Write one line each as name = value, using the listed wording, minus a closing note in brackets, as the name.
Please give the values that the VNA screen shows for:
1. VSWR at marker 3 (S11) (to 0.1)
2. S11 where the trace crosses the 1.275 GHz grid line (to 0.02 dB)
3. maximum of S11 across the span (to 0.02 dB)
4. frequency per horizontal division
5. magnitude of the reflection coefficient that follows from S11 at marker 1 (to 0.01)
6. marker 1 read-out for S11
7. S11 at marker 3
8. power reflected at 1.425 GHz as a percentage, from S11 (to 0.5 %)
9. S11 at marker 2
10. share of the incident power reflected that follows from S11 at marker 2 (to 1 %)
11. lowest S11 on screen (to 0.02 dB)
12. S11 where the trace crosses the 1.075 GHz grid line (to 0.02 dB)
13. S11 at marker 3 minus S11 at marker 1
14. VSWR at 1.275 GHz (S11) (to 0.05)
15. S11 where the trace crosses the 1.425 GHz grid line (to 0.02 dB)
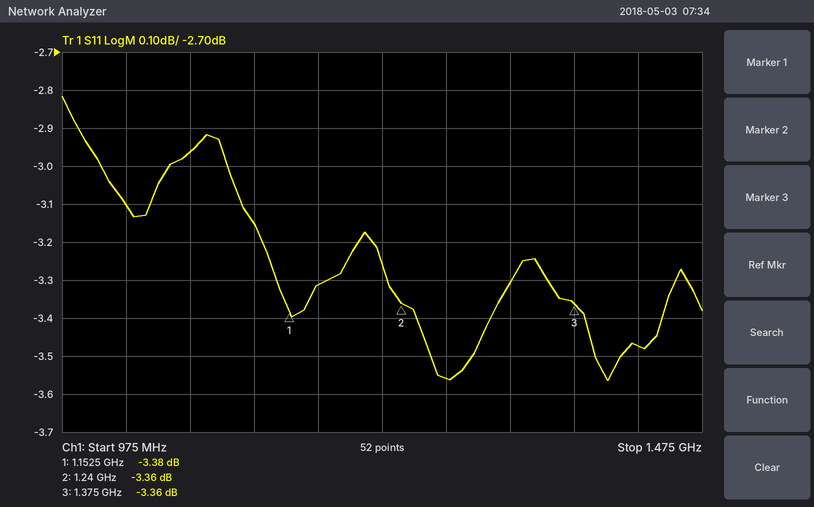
VSWR at marker 3 (S11) = 5.2
S11 where the trace crosses the 1.275 GHz grid line = -3.56 dB
maximum of S11 across the span = -2.82 dB
frequency per horizontal division = 50 MHz
magnitude of the reflection coefficient that follows from S11 at marker 1 = 0.68
marker 1 read-out for S11 = -3.38 dB
S11 at marker 3 = -3.36 dB
power reflected at 1.425 GHz as a percentage, from S11 = 45.0 %
S11 at marker 2 = -3.36 dB
share of the incident power reflected that follows from S11 at marker 2 = 46 %
lowest S11 on screen = -3.56 dB
S11 where the trace crosses the 1.075 GHz grid line = -2.96 dB
S11 at marker 3 minus S11 at marker 1 = 0.02 dB
VSWR at 1.275 GHz (S11) = 4.95
S11 where the trace crosses the 1.425 GHz grid line = -3.48 dB
